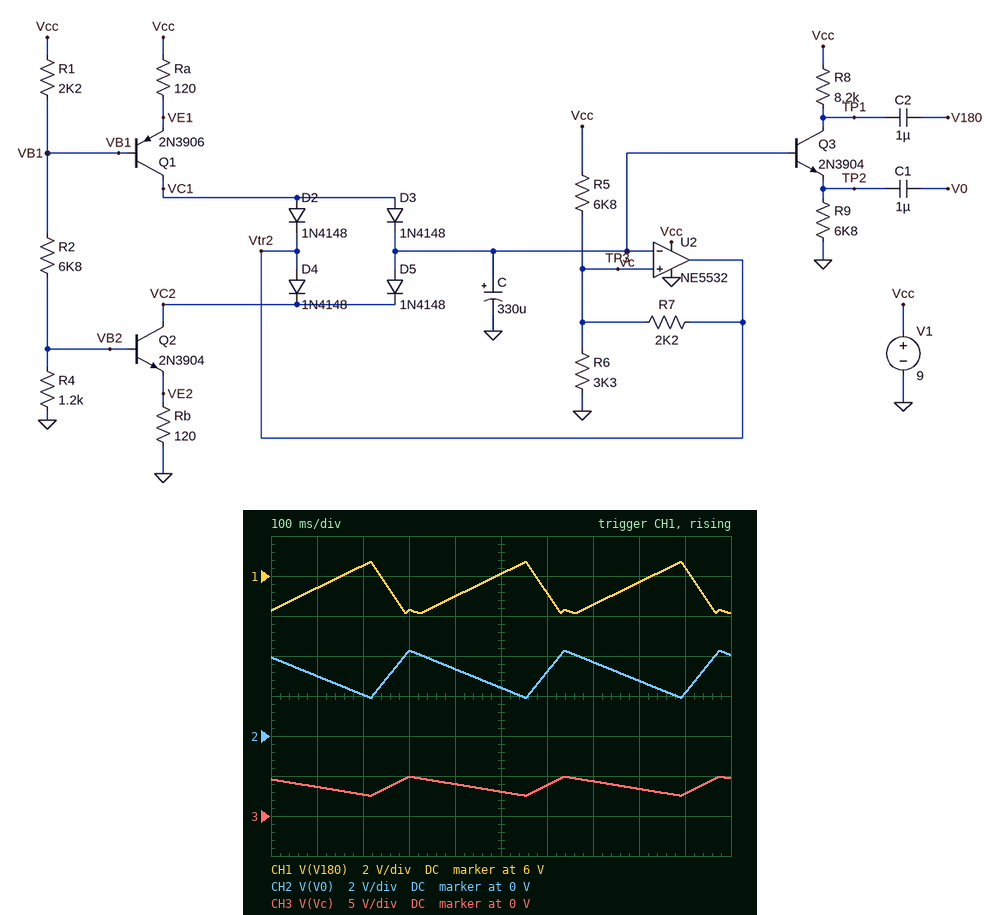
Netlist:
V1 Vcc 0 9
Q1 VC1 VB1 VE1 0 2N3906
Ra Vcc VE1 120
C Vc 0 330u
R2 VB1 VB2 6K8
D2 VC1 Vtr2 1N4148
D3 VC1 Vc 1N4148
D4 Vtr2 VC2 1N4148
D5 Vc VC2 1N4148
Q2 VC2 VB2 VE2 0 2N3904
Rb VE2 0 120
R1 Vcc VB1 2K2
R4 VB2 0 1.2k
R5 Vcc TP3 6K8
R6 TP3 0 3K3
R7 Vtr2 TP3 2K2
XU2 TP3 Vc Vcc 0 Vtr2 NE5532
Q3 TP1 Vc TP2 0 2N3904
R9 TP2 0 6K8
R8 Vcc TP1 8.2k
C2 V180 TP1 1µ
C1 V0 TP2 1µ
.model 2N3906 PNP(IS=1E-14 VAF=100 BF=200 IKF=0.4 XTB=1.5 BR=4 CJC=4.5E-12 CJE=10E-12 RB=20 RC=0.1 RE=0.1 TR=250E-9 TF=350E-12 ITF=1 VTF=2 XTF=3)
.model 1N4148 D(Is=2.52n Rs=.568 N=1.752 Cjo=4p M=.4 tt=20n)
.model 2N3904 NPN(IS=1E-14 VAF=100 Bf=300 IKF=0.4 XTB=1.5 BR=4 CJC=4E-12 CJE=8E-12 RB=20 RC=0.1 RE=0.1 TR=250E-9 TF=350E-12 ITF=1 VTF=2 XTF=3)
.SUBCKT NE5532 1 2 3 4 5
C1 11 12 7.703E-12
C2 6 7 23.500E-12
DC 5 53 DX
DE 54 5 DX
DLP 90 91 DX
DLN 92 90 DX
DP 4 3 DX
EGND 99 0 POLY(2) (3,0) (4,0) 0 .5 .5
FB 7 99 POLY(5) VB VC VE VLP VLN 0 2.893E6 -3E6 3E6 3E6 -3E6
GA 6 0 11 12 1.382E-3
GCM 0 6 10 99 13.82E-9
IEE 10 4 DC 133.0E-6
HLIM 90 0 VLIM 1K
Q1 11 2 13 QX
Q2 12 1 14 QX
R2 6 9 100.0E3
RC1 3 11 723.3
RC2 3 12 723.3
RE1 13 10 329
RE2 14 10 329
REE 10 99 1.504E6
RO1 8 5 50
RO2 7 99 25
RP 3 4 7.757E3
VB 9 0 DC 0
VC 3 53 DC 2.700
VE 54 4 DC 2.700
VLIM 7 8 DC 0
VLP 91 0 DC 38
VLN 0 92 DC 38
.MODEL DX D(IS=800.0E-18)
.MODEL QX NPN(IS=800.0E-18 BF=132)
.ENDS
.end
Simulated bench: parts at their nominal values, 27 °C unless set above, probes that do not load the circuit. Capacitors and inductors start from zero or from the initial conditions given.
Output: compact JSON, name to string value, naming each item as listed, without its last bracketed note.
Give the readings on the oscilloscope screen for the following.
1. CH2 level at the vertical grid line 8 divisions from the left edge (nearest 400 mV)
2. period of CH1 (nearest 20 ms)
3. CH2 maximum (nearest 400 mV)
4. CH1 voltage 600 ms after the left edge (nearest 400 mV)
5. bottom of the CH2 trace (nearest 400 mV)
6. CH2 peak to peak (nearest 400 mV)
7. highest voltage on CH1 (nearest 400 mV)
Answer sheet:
{"CH2 level at the vertical grid line 8 divisions from the left edge": "2.8 V", "period of CH1": "340 ms", "CH2 maximum": "4.4 V", "CH1 voltage 600 ms after the left edge": "5.2 V", "bottom of the CH2 trace": "2.0 V", "CH2 peak to peak": "2.4 V", "highest voltage on CH1": "6.8 V"}
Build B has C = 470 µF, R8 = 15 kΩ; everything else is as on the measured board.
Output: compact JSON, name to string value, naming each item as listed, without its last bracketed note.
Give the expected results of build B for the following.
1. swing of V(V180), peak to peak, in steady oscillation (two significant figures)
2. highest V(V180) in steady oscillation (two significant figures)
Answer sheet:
{"swing of V(V180), peak to peak, in steady oscillation": "1.9 V", "highest V(V180) in steady oscillation": "4.8 V"}
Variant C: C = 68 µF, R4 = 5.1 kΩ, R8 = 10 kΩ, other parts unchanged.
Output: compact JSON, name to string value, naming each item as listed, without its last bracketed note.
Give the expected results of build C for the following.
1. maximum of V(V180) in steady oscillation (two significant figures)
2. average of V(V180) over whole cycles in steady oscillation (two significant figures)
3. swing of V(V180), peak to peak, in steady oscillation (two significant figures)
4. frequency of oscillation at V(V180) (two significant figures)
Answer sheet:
{"maximum of V(V180) in steady oscillation": "6.2 V", "average of V(V180) over whole cycles in steady oscillation": "4.7 V", "swing of V(V180), peak to peak, in steady oscillation": "2.5 V", "frequency of oscillation at V(V180)": "27 Hz"}
